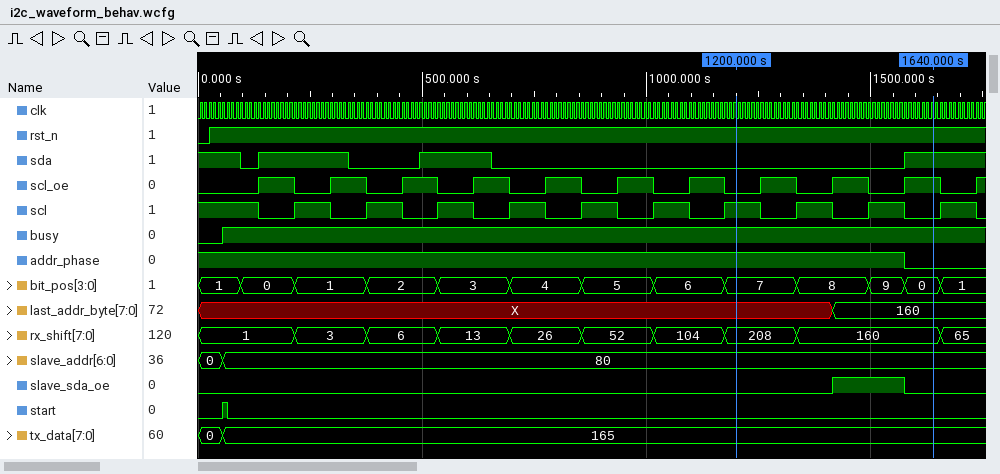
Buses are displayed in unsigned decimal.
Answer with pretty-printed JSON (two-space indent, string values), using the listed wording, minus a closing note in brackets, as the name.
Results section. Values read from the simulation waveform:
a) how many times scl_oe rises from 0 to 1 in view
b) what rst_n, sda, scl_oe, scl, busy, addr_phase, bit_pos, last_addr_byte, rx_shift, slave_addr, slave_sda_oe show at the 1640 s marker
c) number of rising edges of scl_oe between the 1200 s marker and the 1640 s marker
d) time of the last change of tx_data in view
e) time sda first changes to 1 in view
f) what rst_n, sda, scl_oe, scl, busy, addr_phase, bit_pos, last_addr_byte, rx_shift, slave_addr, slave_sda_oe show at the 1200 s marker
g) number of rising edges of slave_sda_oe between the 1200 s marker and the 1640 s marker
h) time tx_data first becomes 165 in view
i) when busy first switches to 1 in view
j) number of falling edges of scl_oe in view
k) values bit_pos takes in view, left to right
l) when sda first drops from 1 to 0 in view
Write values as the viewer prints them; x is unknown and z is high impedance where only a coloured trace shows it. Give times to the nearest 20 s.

{
  "how many times scl_oe rises from 0 to 1 in view": "11",
  "what rst_n, sda, scl_oe, scl, busy, addr_phase, bit_pos, last_addr_byte, rx_shift, slave_addr, slave_sda_oe show at the 1640 s marker": "rst_n=1, sda=1, scl_oe=1, scl=0, busy=1, addr_phase=0, bit_pos=0, last_addr_byte=160, rx_shift=160, slave_addr=80, slave_sda_oe=0",
  "number of rising edges of scl_oe between the 1200 s marker and the 1640 s marker": "3",
  "time of the last change of tx_data in view": "60 s",
  "time sda first changes to 1 in view": "140 s",
  "what rst_n, sda, scl_oe, scl, busy, addr_phase, bit_pos, last_addr_byte, rx_shift, slave_addr, slave_sda_oe show at the 1200 s marker": "rst_n=1, sda=0, scl_oe=0, scl=1, busy=1, addr_phase=1, bit_pos=7, last_addr_byte=X, rx_shift=208, slave_addr=80, slave_sda_oe=0",
  "number of rising edges of slave_sda_oe between the 1200 s marker and the 1640 s marker": "1",
  "time tx_data first becomes 165 in view": "60 s",
  "when busy first switches to 1 in view": "60 s",
  "number of falling edges of scl_oe in view": "10",
  "values bit_pos takes in view, left to right": "1, 0, 1, 2, 3, 4, 5, 6, 7, 8, 9, 0, 1",
  "when sda first drops from 1 to 0 in view": "100 s"
}
